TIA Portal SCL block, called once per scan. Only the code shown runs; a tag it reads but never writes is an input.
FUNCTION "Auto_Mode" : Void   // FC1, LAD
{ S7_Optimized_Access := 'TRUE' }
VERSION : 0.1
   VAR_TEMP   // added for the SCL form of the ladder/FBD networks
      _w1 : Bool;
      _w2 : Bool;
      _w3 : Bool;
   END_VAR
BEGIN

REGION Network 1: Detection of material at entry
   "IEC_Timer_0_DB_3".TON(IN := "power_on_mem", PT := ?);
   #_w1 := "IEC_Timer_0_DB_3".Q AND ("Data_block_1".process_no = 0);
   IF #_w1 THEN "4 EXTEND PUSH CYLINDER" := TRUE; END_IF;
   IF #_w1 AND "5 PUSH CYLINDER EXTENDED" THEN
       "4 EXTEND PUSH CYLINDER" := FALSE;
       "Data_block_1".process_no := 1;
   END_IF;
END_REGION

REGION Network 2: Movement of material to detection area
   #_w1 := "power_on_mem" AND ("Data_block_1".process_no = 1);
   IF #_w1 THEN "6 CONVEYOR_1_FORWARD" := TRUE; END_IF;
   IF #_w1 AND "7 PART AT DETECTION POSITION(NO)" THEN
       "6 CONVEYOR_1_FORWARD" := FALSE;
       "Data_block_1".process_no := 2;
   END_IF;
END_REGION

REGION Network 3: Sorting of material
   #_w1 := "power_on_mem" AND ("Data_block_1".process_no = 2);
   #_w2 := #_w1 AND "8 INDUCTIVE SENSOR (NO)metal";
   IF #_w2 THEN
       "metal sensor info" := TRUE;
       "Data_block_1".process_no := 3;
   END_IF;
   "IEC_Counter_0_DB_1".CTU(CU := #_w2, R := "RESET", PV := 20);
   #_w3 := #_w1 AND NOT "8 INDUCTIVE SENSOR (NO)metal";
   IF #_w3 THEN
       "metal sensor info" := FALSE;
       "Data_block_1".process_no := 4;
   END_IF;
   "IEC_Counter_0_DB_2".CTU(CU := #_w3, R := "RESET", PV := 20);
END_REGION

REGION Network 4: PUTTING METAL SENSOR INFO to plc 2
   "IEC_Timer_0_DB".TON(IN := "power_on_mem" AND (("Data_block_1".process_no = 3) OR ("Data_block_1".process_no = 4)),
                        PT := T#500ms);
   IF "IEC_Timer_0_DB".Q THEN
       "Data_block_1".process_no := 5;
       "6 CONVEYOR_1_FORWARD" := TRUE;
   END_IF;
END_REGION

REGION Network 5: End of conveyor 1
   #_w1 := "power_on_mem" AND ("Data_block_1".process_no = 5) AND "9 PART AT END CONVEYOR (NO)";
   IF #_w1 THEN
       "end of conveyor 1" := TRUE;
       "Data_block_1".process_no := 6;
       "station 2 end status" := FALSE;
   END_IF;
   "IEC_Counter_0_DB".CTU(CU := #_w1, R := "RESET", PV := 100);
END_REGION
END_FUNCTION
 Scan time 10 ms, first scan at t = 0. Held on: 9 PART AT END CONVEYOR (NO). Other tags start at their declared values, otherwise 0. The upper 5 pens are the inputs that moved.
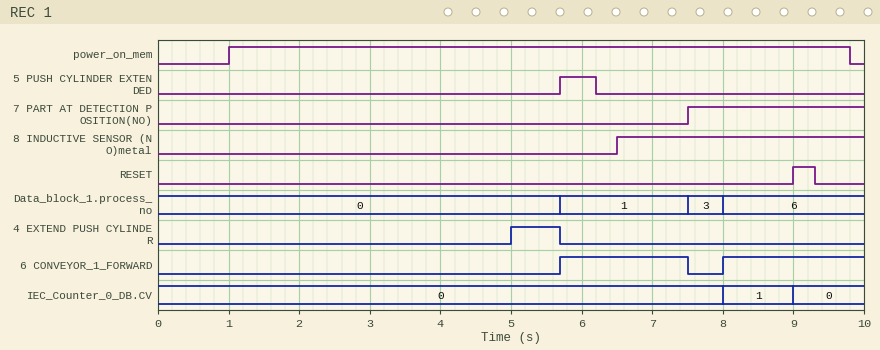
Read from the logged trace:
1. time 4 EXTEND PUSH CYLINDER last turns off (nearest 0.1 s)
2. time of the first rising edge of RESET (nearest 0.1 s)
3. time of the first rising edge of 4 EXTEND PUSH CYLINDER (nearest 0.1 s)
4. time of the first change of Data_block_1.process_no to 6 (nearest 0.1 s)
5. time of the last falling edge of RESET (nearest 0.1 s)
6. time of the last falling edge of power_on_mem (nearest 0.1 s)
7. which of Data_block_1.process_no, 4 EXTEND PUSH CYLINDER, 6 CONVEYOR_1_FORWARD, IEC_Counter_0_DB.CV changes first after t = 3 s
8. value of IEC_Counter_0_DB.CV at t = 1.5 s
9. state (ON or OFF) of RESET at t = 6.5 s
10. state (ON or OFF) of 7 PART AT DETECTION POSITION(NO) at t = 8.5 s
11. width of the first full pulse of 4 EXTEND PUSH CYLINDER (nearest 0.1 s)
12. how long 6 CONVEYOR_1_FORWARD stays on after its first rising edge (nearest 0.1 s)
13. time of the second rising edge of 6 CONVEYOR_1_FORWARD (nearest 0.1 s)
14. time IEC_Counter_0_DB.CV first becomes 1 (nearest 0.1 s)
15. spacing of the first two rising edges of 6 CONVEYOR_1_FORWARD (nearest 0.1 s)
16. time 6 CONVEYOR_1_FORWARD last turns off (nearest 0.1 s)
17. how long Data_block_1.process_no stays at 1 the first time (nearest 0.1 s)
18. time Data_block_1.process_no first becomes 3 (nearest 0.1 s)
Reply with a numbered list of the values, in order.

1. 5.7 s
2. 9.0 s
3. 5.0 s
4. 8.0 s
5. 9.3 s
6. 9.8 s
7. 4 EXTEND PUSH CYLINDER
8. 0
9. OFF
10. ON
11. 0.7 s
12. 1.8 s
13. 8.0 s
14. 8.0 s
15. 2.3 s
16. 7.5 s
17. 1.8 s
18. 7.5 s
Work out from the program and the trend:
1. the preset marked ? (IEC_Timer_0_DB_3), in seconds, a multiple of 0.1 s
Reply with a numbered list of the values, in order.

1. 4.0 s
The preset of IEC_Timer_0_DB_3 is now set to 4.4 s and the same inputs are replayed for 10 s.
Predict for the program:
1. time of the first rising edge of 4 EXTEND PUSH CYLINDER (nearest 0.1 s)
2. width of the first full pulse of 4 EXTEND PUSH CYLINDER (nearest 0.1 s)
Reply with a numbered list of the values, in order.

1. 5.4 s
2. 0.3 s
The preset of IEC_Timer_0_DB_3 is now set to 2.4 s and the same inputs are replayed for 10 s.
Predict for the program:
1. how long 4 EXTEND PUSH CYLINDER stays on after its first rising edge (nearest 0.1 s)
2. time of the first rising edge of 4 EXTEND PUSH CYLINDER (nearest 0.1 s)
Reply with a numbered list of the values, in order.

1. 2.3 s
2. 3.4 s
